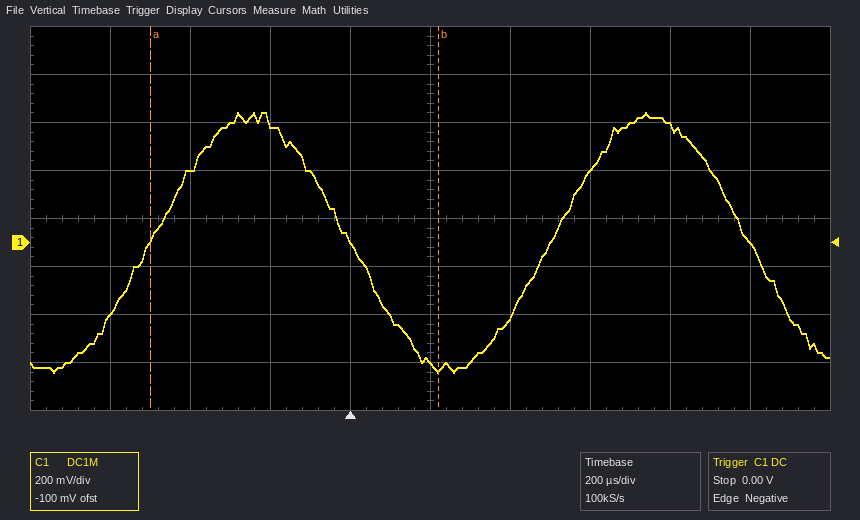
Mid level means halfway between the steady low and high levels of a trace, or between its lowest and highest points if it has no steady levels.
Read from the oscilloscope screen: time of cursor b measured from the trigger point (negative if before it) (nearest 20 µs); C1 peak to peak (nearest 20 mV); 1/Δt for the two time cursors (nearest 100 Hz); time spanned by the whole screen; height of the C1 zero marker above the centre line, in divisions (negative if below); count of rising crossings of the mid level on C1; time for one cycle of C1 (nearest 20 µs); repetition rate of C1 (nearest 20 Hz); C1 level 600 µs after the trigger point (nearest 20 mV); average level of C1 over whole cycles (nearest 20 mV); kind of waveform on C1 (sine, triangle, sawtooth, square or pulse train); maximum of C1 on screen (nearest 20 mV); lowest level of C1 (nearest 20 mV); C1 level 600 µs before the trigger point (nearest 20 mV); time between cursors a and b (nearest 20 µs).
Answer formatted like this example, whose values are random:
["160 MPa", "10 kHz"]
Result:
["+220 µs", "1.08 V", "1.4 kHz", "2 ms", "-0.5 div", "2", "1.00 ms", "1.00 kHz", "300 mV", "0 mV", "sine", "540 mV", "-540 mV", "-300 mV", "720 µs"]
